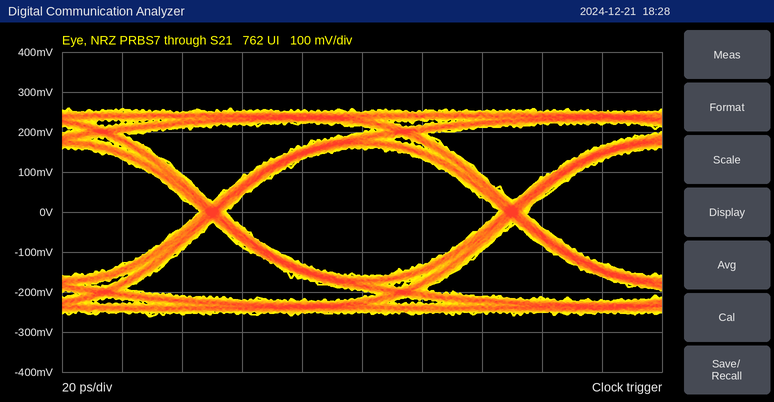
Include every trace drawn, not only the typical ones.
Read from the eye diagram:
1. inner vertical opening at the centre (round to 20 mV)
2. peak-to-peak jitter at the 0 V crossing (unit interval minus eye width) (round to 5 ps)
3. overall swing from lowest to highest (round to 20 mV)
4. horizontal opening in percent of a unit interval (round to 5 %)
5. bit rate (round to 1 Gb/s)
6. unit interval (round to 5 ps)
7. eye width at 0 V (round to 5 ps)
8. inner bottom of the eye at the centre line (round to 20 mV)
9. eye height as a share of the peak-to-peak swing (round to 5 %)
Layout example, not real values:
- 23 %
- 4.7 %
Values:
- 320 mV
- 10 ps
- 520 mV
- 90 %
- 10 Gb/s
- 100 ps
- 90 ps
- -160 mV
- 60 %
